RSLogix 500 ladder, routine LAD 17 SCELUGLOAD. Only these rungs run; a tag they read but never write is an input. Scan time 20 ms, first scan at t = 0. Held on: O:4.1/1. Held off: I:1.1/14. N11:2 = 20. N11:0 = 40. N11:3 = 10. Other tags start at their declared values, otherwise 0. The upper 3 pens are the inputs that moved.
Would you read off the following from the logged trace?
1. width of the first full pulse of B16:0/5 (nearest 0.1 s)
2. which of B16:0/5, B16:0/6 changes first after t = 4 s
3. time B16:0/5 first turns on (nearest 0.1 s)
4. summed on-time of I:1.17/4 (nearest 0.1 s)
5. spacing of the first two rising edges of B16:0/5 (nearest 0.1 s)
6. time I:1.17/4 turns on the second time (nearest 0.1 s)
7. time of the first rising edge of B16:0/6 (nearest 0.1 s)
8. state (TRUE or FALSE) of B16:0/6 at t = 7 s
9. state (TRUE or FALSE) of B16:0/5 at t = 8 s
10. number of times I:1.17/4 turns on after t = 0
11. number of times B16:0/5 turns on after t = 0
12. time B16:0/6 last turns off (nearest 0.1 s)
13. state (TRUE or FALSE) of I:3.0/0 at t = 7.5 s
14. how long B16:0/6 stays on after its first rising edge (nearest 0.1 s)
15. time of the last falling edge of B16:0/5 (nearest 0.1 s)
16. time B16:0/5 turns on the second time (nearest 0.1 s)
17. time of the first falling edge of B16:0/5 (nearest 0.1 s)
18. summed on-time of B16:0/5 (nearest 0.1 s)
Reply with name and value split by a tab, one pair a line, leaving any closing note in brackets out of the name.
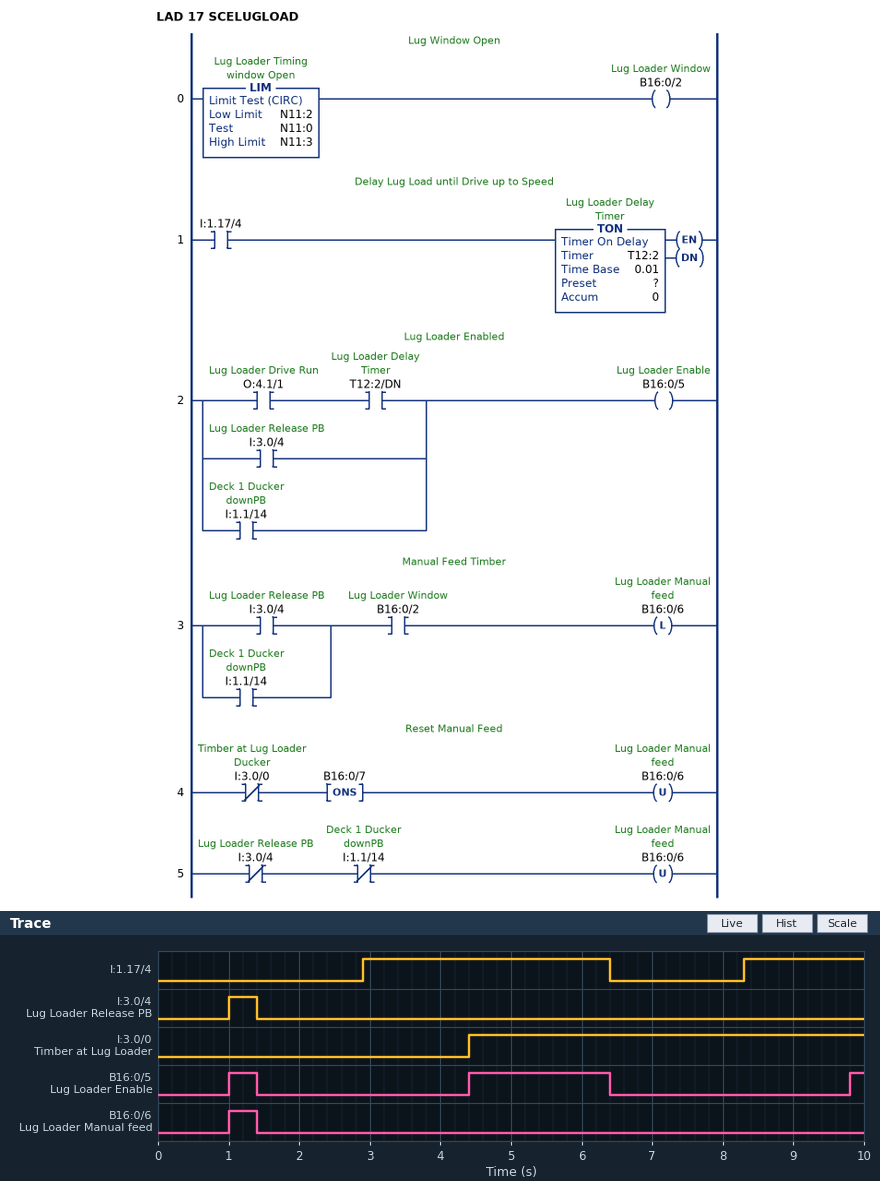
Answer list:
width of the first full pulse of B16:0/5	0.4 s
which of B16:0/5, B16:0/6 changes first after t = 4 s	B16:0/5
time B16:0/5 first turns on	1.0 s
summed on-time of I:1.17/4	5.2 s
spacing of the first two rising edges of B16:0/5	3.4 s
time I:1.17/4 turns on the second time	8.3 s
time of the first rising edge of B16:0/6	1.0 s
state (TRUE or FALSE) of B16:0/6 at t = 7 s	FALSE
state (TRUE or FALSE) of B16:0/5 at t = 8 s	FALSE
number of times I:1.17/4 turns on after t = 0	2
number of times B16:0/5 turns on after t = 0	3
time B16:0/6 last turns off	1.4 s
state (TRUE or FALSE) of I:3.0/0 at t = 7.5 s	TRUE
how long B16:0/6 stays on after its first rising edge	0.4 s
time of the last falling edge of B16:0/5	6.4 s
time B16:0/5 turns on the second time	4.4 s
time of the first falling edge of B16:0/5	1.4 s
summed on-time of B16:0/5	2.6 s
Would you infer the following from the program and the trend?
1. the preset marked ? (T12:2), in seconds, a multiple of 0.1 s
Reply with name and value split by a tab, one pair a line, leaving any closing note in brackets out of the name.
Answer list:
the preset marked ? (T12:2), in seconds, a multiple of 0.1 s	1.5 s
